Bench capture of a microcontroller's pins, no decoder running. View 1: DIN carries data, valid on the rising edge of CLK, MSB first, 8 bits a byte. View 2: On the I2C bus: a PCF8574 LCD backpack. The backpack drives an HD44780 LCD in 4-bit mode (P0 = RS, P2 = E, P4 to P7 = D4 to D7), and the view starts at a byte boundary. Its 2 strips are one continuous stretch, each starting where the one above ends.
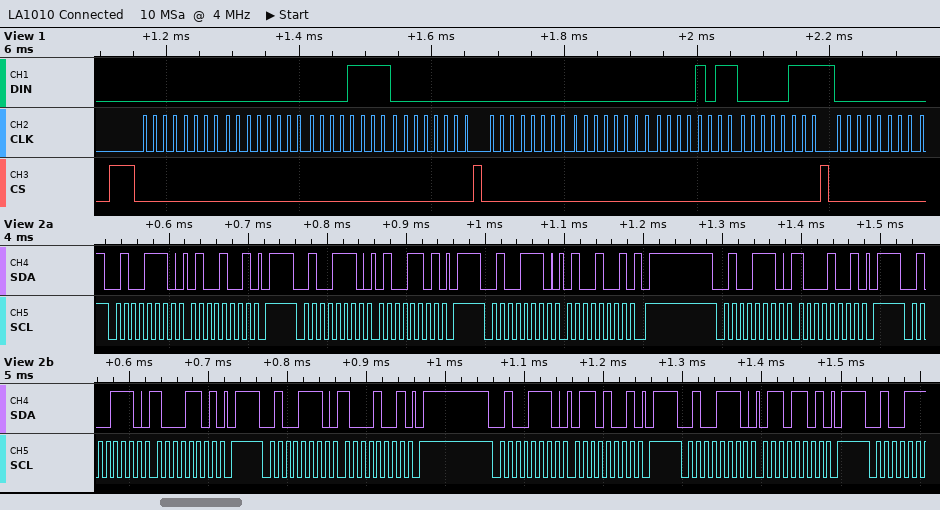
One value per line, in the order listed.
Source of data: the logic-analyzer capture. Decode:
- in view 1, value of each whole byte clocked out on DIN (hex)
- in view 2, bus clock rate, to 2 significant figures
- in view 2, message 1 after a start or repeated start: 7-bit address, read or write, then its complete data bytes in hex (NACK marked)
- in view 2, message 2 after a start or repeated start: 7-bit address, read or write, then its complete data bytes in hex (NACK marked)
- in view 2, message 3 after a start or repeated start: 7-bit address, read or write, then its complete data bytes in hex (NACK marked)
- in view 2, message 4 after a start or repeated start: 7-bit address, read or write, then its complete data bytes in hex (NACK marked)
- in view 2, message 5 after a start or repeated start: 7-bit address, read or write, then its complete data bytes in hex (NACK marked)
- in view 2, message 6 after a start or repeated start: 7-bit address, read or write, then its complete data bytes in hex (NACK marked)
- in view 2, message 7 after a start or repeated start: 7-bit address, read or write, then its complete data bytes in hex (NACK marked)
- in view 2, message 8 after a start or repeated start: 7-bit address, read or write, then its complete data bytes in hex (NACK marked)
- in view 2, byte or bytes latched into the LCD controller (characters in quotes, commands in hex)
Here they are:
0x00 0x00 0x0F 0x00 0x00 0x00 0x0B 0x07 0x00
100 kHz
0x27 write: 49
0x27 write: 4D
0x27 write: 49
0x27 write: 89
0x27 write: 8D
0x27 write: 89
0x27 write: 69
0x27 write: 6D
'H'
